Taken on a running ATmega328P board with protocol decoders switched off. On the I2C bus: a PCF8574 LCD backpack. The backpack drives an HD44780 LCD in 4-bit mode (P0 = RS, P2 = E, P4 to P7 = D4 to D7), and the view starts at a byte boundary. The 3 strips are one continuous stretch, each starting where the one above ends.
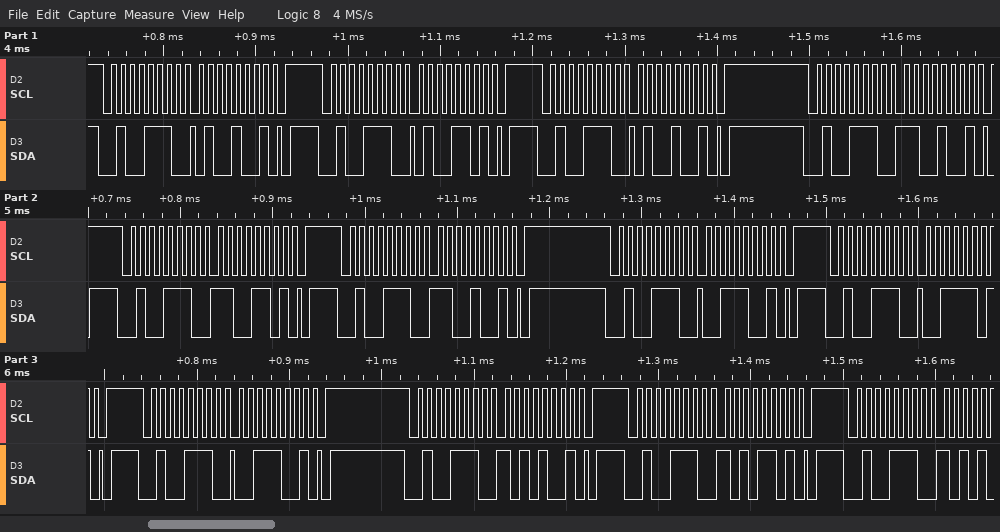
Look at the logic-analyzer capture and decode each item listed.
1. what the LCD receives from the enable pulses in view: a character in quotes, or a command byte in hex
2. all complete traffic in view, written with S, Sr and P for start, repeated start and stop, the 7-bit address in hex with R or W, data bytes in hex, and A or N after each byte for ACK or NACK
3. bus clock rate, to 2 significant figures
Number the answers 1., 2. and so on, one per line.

1. 'L'
2. S 27W A 49 A P S 27W A 4D A P S 27W A 49 A P S 27W A C9 A P S 27W A CD A P S 27W A C9 A P S 27W A 39 A P S 27W A 3D A P S 27W A 39 A P S 27W A A9 A P S 27W A AD A P S 27W A
3. 100 kHz
